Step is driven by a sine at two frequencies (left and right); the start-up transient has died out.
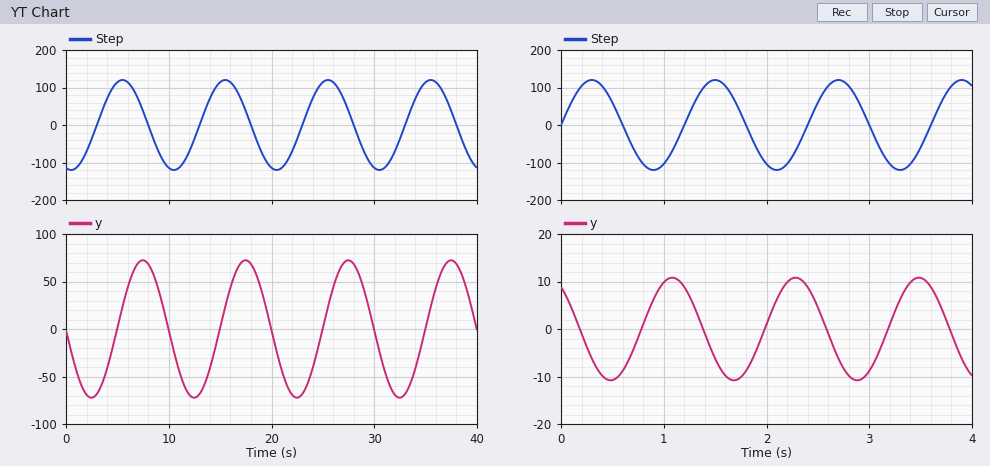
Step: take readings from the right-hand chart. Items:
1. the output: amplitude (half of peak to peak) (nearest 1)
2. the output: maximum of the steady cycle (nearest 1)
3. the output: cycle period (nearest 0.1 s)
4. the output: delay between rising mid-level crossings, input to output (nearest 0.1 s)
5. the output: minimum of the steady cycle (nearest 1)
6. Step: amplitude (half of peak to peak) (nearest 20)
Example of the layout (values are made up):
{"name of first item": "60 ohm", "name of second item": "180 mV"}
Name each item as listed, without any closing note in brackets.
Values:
{"the output: amplitude (half of peak to peak)": "11", "the output: maximum of the steady cycle": "11", "the output: cycle period": "1.2 s", "the output: delay between rising mid-level crossings, input to output": "0.8 s", "the output: minimum of the steady cycle": "-11", "Step: amplitude (half of peak to peak)": "120"}
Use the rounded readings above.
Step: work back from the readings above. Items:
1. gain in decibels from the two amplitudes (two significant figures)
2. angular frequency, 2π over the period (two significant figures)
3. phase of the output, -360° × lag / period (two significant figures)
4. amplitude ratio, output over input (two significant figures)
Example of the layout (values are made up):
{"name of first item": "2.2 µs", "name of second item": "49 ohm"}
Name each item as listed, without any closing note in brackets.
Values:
{"gain in decibels from the two amplitudes": "-21 dB", "angular frequency, 2π over the period": "5.2 rad/s", "phase of the output, -360° × lag / period": "-240°", "amplitude ratio, output over input": "0.092"}
